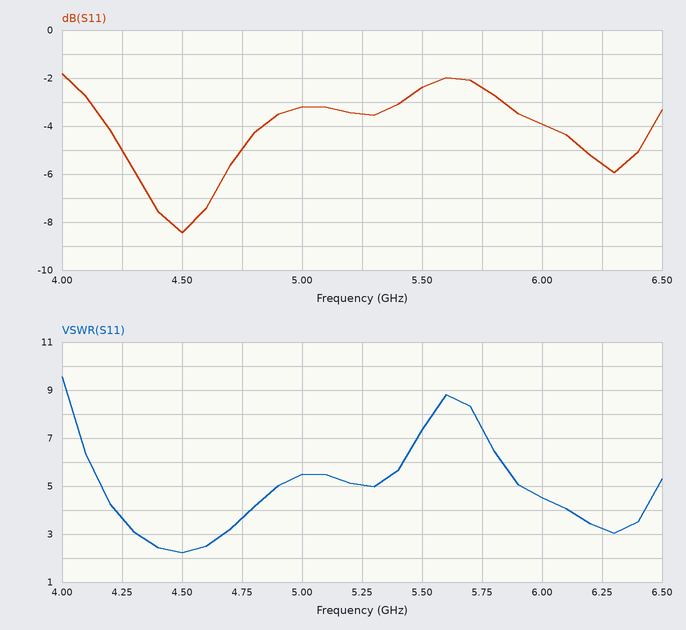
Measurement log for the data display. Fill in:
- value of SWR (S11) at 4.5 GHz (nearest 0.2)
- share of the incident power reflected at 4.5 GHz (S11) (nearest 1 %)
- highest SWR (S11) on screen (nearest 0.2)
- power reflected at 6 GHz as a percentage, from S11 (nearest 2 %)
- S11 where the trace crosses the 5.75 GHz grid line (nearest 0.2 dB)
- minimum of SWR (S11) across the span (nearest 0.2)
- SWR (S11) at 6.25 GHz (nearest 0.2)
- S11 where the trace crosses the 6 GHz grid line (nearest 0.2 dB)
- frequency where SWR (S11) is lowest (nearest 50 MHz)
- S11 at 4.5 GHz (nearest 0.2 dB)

2.2
14 %
9.6
40 %
-2.4 dB
2.2
3.2
-4.0 dB
4.50 GHz
-8.4 dB
